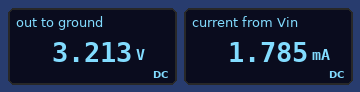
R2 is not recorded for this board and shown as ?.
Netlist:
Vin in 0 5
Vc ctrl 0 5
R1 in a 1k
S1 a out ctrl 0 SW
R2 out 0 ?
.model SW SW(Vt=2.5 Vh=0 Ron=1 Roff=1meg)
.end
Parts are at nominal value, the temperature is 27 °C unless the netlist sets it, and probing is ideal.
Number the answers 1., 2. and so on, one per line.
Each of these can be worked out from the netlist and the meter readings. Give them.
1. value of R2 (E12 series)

1. 1.8 kΩ
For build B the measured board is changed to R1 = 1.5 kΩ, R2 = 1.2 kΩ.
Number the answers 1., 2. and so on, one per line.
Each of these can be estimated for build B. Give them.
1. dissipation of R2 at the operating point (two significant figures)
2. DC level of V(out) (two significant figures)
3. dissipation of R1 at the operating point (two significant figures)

1. 4.1 mW
2. 2.2 V
3. 5.1 mW
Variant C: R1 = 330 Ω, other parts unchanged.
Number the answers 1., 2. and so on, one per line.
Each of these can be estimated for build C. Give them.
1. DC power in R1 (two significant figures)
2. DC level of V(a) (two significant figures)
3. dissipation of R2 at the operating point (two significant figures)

1. 1.8 mW
2. 4.2 V
3. 9.9 mW
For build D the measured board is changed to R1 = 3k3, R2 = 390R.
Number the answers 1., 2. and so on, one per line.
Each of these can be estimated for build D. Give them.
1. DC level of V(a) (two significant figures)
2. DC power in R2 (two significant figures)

1. 530 mV
2. 720 µW
